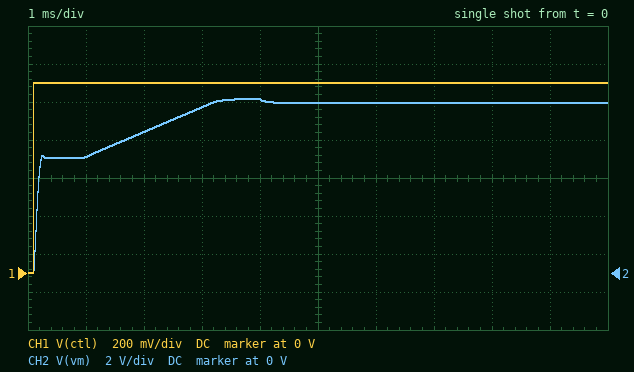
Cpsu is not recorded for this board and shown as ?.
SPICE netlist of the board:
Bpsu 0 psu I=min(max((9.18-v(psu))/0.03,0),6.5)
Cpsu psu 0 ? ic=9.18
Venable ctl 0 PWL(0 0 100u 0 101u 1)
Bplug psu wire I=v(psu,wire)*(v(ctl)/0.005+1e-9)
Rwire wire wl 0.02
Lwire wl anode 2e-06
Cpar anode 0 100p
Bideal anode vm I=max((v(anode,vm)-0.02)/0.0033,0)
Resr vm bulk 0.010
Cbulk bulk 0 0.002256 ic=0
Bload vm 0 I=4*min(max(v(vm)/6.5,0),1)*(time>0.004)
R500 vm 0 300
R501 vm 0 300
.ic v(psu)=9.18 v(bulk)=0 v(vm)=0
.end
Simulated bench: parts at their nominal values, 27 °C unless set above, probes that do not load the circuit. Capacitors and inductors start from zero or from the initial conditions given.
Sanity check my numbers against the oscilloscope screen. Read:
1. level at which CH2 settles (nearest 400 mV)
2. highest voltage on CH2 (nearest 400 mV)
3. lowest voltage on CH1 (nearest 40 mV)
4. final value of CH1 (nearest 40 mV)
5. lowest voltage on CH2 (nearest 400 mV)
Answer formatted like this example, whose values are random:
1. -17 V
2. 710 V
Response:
1. 8.8 V
2. 9.2 V
3. 0 V
4. 1.00 V
5. 0 V
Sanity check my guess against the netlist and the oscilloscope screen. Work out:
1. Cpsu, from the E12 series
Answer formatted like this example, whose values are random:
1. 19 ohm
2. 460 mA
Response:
1. 2.7 mF
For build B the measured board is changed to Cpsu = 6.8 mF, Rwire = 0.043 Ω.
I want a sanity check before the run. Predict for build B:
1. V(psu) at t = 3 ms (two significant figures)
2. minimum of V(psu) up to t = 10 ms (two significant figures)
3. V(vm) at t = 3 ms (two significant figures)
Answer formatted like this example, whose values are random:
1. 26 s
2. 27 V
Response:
1. 9.0 V
2. 7.1 V
3. 8.9 V
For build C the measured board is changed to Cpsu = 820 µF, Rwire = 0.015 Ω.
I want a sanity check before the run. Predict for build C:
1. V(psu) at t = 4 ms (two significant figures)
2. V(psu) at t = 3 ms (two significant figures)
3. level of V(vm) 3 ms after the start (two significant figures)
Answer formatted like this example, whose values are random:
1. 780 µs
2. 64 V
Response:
1. 9.2 V
2. 8.7 V
3. 8.5 V
